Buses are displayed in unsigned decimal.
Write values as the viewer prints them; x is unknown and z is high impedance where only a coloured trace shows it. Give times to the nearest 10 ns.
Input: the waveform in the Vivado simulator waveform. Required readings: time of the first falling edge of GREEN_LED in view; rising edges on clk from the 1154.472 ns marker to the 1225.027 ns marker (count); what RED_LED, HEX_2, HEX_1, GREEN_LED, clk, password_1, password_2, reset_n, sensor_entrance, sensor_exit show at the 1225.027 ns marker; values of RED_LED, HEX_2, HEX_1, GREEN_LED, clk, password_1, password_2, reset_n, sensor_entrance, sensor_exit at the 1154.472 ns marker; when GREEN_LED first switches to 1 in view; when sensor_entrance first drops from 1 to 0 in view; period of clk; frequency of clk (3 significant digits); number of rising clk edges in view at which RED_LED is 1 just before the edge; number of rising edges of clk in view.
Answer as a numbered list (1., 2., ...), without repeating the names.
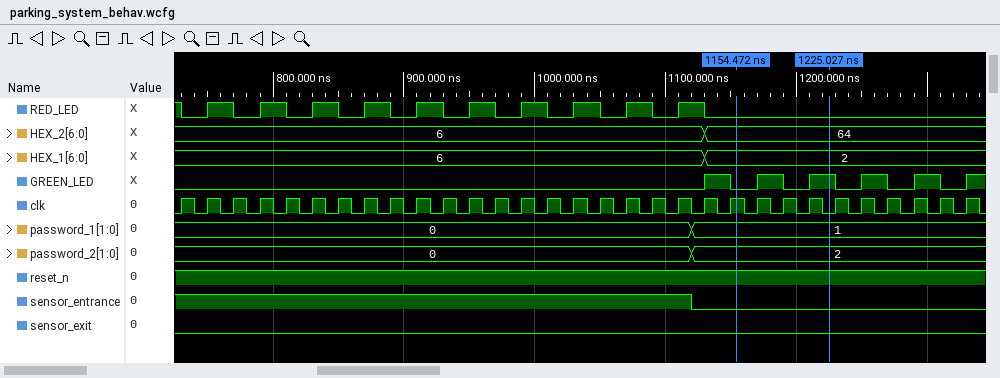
1. 1150 ns
2. 3
3. RED_LED=0, HEX_2=64, HEX_1=2, GREEN_LED=1, clk=0, password_1=1, password_2=2, reset_n=1, sensor_entrance=0, sensor_exit=0
4. RED_LED=0, HEX_2=64, HEX_1=2, GREEN_LED=0, clk=1, password_1=1, password_2=2, reset_n=1, sensor_entrance=0, sensor_exit=0
5. 1130 ns
6. 1120 ns
7. 20 ns
8. 50.0 MHz
9. 11
10. 31
